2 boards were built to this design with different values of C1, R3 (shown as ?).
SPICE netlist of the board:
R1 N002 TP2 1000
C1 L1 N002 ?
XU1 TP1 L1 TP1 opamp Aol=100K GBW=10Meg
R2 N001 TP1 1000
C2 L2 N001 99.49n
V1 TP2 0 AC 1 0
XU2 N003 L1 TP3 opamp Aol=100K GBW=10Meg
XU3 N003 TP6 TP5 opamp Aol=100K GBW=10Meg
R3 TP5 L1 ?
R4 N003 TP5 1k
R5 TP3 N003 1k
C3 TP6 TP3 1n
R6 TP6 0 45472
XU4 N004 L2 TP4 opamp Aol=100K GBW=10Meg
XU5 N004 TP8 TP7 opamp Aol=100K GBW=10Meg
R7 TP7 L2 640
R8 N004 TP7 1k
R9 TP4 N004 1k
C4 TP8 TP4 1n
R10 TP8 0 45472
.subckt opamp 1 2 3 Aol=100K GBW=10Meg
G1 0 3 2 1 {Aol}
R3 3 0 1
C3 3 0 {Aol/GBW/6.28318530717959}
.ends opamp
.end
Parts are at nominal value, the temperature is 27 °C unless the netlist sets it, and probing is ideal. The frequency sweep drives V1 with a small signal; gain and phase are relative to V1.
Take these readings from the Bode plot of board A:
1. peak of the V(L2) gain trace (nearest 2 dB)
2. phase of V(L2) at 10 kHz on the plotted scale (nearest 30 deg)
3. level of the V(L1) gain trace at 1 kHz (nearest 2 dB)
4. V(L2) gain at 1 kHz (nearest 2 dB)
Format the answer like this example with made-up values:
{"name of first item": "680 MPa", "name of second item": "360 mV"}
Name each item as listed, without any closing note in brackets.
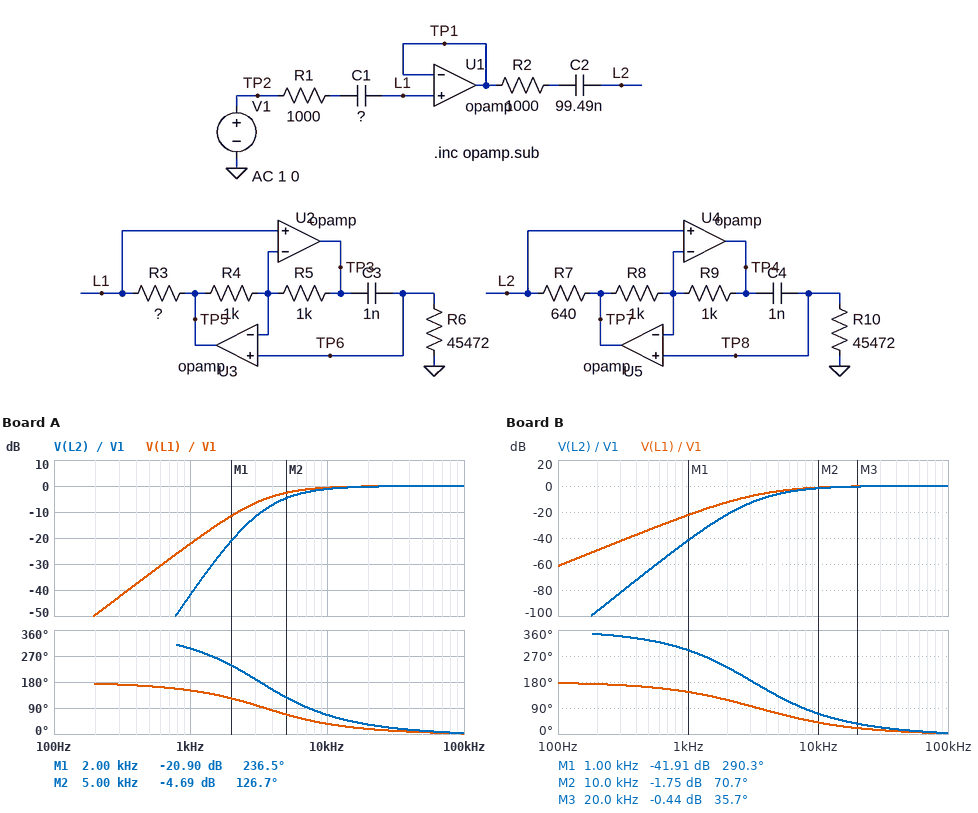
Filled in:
{"peak of the V(L2) gain trace": "0 dB", "phase of V(L2) at 10 kHz on the plotted scale": "60 deg", "level of the V(L1) gain trace at 1 kHz": "-22 dB", "V(L2) gain at 1 kHz": "-42 dB"}
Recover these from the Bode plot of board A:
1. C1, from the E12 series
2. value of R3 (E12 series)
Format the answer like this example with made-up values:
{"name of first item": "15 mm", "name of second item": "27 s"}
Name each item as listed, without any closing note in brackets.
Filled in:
{"C1, from the E12 series": "82 nF", "value of R3": "560 Ω"}
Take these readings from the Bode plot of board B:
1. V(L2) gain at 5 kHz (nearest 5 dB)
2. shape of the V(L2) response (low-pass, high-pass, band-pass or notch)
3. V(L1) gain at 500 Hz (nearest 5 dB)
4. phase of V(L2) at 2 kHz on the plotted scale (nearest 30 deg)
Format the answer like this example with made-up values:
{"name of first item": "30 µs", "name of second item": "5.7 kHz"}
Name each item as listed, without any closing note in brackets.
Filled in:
{"V(L2) gain at 5 kHz": "-5 dB", "shape of the V(L2) response": "high-pass", "V(L1) gain at 500 Hz": "-35 dB", "phase of V(L2) at 2 kHz on the plotted scale": "240 deg"}
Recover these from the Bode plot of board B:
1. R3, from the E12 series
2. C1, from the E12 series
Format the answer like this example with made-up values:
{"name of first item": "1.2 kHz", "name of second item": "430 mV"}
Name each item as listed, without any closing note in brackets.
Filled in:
{"R3, from the E12 series": "470 Ω", "C1, from the E12 series": "100 nF"}
